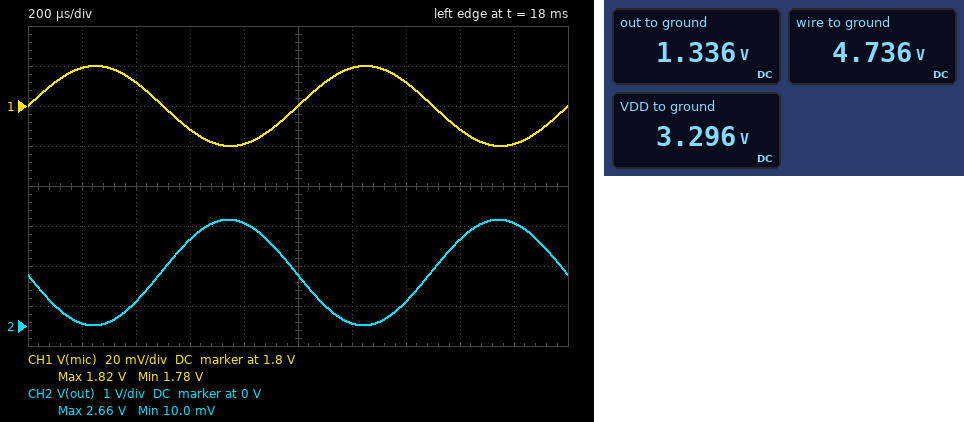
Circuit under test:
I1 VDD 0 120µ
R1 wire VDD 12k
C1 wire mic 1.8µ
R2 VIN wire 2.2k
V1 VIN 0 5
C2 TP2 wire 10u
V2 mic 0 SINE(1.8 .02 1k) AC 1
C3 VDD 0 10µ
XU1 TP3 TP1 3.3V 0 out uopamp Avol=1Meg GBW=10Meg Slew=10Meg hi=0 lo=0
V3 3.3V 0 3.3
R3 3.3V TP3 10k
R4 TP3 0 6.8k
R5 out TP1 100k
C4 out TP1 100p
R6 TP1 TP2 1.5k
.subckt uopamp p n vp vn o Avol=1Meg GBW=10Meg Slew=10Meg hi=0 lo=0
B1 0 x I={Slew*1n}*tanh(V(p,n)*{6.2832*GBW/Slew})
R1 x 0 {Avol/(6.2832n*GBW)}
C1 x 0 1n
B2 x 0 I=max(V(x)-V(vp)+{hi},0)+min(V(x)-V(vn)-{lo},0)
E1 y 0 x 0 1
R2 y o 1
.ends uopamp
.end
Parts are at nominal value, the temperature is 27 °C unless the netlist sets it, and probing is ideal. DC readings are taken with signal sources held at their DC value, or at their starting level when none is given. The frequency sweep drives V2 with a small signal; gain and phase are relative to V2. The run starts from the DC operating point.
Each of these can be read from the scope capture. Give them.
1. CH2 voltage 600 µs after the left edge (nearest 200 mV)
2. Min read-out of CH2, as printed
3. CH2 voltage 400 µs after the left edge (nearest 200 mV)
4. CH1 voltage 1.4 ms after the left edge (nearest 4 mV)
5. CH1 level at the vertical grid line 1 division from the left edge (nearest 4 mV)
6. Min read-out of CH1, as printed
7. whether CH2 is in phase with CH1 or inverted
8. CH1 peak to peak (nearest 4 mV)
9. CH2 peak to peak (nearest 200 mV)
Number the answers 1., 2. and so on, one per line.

1. 2.2 V
2. 10.0 mV
3. 600 mV
4. 1.812 V
5. 1.820 V
6. 1.78 V
7. inverted
8. 40 mV
9. 2.6 V
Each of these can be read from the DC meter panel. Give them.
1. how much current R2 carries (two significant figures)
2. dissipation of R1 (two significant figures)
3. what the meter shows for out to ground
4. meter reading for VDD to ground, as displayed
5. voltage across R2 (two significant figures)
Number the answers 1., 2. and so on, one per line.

1. 120 µA
2. 170 µW
3. 1.336 V
4. 3.296 V
5. 260 mV
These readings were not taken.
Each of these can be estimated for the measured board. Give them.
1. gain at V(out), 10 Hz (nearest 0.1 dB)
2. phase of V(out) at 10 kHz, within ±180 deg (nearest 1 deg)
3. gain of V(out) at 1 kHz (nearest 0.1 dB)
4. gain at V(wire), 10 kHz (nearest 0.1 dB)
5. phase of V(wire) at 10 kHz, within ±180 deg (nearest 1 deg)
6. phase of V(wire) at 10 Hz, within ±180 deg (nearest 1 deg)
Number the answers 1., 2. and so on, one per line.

1. 14.6 dB
2. 146 deg
3. 36.4 dB
4. 0 dB
5. 1 deg
6. 62 deg
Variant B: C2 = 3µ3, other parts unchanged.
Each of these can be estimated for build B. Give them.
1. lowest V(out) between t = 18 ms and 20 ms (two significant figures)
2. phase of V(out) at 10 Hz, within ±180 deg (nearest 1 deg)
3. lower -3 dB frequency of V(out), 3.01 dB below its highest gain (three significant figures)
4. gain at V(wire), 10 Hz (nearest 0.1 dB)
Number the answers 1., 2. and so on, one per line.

1. 15 mV
2. -45 deg
3. 126 Hz
4. -15.5 dB
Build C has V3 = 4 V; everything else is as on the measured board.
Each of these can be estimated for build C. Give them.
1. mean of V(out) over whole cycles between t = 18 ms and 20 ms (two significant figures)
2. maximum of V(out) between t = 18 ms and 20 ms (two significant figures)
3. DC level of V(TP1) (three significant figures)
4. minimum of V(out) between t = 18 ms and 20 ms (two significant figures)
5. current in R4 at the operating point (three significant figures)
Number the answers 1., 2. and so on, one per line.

1. 1.6 V
2. 2.9 V
3. 1.62 V
4. 300 mV
5. 238 µA
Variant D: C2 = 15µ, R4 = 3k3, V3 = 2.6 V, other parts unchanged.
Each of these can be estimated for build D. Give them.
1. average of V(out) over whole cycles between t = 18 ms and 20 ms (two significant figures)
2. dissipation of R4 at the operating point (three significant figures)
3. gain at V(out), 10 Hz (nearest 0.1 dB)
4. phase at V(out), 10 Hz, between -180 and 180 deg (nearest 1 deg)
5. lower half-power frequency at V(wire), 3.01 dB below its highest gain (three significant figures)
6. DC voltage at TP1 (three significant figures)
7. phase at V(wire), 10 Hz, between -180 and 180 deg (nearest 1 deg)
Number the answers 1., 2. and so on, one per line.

1. 710 mV
2. 126 µW
3. 15.2 dB
4. -79 deg
5. 110 Hz
6. 645 mV
7. 66 deg
